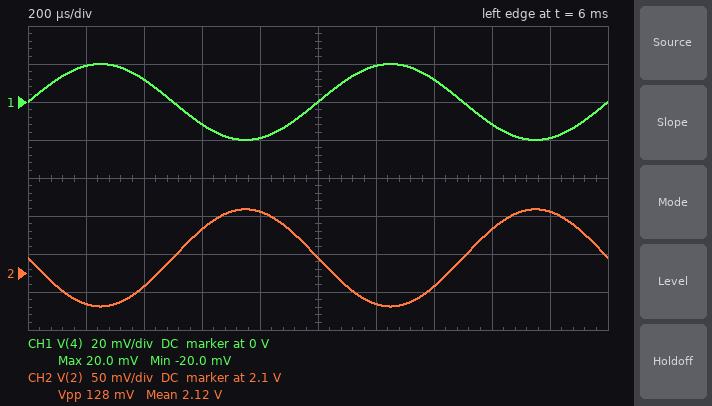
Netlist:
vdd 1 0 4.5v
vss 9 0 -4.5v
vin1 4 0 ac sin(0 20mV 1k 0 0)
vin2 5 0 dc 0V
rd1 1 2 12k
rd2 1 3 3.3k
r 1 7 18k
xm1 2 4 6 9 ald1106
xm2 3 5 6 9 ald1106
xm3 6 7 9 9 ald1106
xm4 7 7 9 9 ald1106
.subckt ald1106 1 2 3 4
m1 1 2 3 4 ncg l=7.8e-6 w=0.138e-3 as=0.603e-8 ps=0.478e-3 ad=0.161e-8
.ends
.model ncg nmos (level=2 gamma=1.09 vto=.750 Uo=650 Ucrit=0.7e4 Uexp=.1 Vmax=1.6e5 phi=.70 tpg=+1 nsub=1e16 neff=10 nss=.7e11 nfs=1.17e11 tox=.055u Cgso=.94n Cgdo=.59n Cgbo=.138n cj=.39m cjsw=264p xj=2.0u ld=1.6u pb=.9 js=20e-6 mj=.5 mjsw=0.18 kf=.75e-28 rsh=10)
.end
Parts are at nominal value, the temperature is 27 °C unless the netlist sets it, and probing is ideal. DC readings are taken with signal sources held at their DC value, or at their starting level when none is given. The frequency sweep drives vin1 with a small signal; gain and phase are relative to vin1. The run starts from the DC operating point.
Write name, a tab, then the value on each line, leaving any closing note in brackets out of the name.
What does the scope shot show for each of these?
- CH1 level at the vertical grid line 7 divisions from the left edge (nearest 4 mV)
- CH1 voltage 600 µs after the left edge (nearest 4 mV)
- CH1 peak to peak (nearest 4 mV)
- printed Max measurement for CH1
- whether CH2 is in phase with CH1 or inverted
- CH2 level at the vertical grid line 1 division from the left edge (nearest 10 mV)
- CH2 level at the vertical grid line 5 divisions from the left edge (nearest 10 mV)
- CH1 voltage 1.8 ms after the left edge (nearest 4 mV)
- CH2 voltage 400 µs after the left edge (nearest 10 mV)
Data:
CH1 level at the vertical grid line 7 divisions from the left edge	12 mV
CH1 voltage 600 µs after the left edge	-12 mV
CH1 peak to peak	40 mV
printed Max measurement for CH1	20.0 mV
whether CH2 is in phase with CH1 or inverted	inverted
CH2 level at the vertical grid line 1 division from the left edge	2.06 V
CH2 level at the vertical grid line 5 divisions from the left edge	2.12 V
CH1 voltage 1.8 ms after the left edge	-20 mV
CH2 voltage 400 µs after the left edge	2.08 V
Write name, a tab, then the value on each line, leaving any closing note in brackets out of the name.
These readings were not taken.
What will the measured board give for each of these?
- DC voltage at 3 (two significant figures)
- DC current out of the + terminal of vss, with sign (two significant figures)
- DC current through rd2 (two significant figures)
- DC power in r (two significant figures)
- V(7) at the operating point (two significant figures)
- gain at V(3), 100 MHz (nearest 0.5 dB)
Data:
DC voltage at 3	3.8 V
DC current out of the + terminal of vss, with sign	-810 µA
DC current through rd2	210 µA
DC power in r	2.9 mW
V(7) at the operating point	-2.7 V
gain at V(3), 100 MHz	-7.5 dB
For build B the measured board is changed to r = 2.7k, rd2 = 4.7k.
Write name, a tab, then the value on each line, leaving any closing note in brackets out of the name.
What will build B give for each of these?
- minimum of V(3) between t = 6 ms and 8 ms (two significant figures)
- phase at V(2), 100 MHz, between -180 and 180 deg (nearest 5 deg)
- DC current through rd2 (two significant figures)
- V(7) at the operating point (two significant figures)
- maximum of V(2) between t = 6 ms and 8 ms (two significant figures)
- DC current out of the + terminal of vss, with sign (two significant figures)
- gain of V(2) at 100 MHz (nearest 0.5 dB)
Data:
minimum of V(3) between t = 6 ms and 8 ms	-1.6 V
phase at V(2), 100 MHz, between -180 and 180 deg	105 deg
DC current through rd2	1.3 mA
V(7) at the operating point	-1.2 V
maximum of V(2) between t = 6 ms and 8 ms	-2.7 V
DC current out of the + terminal of vss, with sign	-4.0 mA
gain of V(2) at 100 MHz	-14.5 dB
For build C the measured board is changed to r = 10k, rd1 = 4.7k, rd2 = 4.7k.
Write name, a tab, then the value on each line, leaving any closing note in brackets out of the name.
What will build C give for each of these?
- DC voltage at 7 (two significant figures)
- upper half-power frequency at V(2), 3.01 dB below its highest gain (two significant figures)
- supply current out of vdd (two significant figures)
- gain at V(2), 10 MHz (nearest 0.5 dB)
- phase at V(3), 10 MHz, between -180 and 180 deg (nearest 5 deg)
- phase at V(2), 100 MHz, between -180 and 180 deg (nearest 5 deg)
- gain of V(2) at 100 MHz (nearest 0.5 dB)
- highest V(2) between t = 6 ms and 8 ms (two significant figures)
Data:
DC voltage at 7	-2.4 V
upper half-power frequency at V(2), 3.01 dB below its highest gain	200 MHz
supply current out of vdd	1.4 mA
gain at V(2), 10 MHz	4.5 dB
phase at V(3), 10 MHz, between -180 and 180 deg	-10 deg
phase at V(2), 100 MHz, between -180 and 180 deg	150 deg
gain of V(2) at 100 MHz	5.5 dB
highest V(2) between t = 6 ms and 8 ms	2.9 V
